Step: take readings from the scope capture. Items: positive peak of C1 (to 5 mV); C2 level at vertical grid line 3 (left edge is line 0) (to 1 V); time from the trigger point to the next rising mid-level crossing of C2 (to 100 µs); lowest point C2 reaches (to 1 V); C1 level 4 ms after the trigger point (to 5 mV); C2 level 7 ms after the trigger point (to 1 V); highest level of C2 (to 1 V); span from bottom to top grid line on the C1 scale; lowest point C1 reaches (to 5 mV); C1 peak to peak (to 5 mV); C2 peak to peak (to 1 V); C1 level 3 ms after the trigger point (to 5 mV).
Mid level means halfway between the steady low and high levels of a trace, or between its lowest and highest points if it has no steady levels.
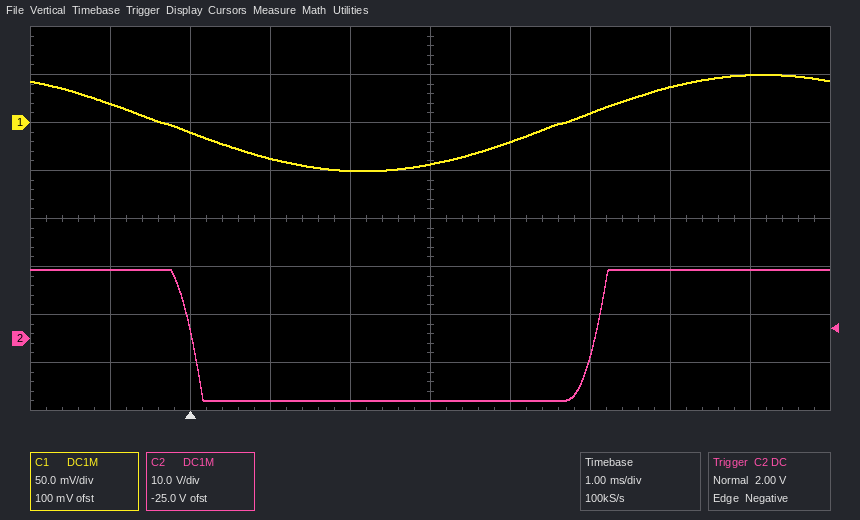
50 mV
-13 V
5.1 ms
-13 V
-20 mV
14 V
14 V
400 mV
-50 mV
100 mV
27 V
-45 mV
